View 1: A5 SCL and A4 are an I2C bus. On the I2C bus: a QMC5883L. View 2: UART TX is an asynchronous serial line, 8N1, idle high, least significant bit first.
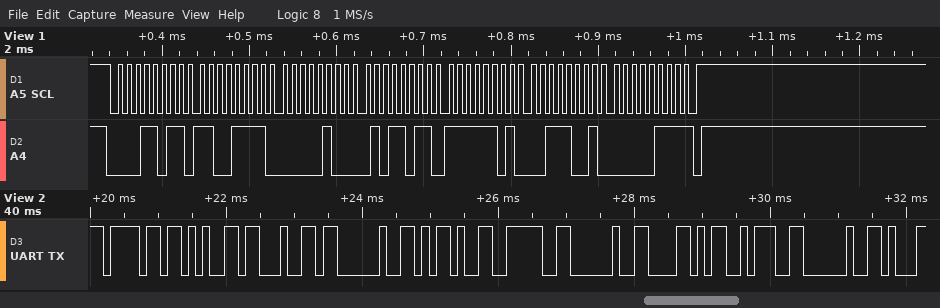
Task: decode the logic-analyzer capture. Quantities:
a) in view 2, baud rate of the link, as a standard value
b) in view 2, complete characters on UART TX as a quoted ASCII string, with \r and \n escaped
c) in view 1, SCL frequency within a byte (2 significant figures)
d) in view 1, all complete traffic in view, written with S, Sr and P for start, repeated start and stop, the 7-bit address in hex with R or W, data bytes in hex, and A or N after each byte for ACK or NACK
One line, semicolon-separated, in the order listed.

9600 baud; "oed -> X: "; 100 kHz; S 0DR A CF A 04 A 5B A FD A 39 A 07 N P
